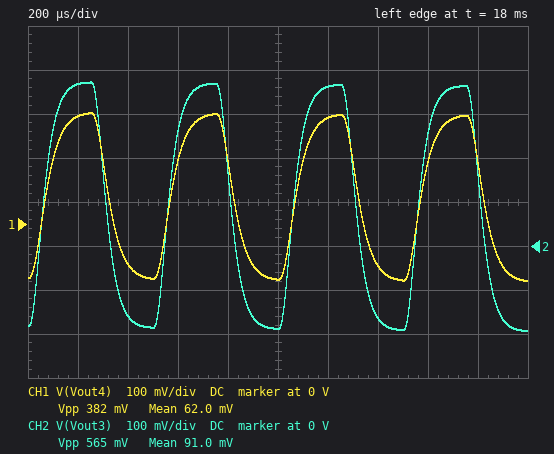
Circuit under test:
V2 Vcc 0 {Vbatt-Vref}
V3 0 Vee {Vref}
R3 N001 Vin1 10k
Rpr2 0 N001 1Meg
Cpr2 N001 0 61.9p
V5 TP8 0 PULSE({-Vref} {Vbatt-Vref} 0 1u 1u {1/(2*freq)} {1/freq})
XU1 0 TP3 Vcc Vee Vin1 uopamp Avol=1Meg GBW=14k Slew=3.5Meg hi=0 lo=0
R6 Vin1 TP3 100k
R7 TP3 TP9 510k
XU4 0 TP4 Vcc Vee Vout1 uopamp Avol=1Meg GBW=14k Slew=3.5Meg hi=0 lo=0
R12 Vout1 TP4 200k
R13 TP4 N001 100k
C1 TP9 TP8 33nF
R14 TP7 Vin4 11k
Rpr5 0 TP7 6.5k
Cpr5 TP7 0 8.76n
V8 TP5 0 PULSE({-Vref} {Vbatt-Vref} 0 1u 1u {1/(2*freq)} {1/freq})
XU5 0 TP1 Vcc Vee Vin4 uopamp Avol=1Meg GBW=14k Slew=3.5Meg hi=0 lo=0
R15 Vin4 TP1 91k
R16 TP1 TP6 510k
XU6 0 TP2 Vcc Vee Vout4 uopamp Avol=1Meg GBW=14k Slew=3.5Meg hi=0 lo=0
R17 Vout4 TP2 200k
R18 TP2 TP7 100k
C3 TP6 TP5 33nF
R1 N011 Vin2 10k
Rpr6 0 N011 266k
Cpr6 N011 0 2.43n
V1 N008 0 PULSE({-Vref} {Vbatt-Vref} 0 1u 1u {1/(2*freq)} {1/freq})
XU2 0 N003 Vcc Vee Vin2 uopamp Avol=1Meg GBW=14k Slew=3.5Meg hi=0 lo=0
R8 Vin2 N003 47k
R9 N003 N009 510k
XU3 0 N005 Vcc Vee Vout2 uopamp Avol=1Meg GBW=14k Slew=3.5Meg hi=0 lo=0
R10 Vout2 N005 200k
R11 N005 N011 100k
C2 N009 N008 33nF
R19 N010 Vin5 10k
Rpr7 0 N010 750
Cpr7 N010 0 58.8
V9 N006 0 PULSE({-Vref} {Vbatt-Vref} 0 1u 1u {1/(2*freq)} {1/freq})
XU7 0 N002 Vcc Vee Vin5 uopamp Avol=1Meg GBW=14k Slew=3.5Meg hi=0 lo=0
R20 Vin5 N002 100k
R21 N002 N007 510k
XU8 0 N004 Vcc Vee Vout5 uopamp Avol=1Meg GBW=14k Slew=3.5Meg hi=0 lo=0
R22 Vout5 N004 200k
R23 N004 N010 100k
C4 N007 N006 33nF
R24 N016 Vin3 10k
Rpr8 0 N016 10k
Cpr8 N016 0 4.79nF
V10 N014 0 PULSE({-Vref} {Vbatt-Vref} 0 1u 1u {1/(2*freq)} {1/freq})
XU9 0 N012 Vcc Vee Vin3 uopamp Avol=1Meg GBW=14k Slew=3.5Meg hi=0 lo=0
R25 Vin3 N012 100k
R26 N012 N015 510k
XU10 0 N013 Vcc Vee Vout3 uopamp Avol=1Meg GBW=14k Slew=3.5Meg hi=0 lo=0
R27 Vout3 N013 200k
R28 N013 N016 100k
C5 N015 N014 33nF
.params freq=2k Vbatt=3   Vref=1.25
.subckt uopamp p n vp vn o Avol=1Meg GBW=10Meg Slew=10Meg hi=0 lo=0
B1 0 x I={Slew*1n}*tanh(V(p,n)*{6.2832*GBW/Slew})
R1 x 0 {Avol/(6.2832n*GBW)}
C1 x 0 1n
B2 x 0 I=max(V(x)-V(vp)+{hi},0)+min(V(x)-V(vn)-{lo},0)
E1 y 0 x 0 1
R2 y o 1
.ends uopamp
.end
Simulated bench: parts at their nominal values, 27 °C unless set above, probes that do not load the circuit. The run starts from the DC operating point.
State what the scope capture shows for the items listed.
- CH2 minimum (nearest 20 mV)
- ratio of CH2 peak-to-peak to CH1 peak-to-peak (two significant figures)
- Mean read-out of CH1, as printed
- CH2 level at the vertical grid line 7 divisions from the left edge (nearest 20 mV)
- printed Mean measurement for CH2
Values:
-200 mV
1.5
62.0 mV
-160 mV
91.0 mV
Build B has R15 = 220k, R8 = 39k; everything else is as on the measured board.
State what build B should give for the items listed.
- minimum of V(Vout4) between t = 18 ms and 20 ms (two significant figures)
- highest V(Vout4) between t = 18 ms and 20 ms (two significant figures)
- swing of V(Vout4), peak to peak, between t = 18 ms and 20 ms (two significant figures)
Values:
-310 mV
610 mV
920 mV
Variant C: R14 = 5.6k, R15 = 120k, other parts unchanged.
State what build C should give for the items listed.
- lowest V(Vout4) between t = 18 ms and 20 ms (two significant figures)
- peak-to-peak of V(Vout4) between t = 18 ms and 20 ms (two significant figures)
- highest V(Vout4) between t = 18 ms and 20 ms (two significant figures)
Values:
-250 mV
740 mV
490 mV
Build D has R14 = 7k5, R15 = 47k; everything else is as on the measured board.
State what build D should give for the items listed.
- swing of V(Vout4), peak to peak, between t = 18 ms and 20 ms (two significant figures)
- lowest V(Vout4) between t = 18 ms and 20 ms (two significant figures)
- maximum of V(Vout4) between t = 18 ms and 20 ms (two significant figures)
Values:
250 mV
-85 mV
160 mV
